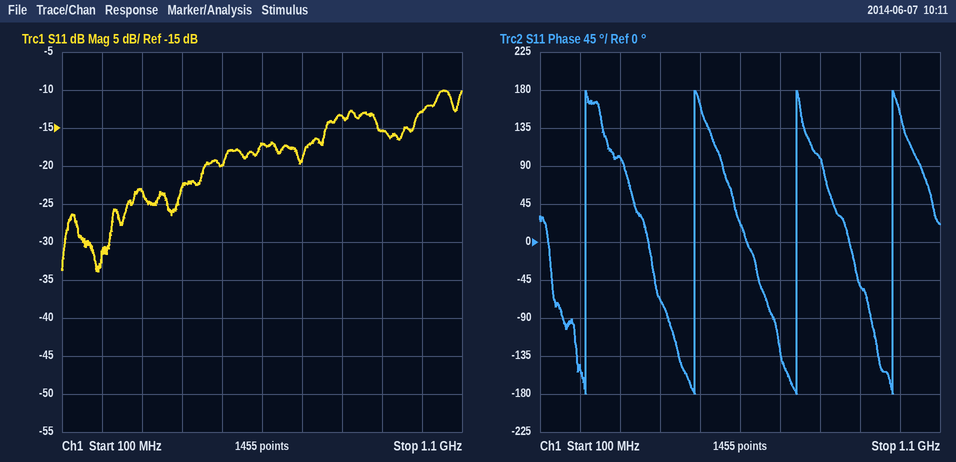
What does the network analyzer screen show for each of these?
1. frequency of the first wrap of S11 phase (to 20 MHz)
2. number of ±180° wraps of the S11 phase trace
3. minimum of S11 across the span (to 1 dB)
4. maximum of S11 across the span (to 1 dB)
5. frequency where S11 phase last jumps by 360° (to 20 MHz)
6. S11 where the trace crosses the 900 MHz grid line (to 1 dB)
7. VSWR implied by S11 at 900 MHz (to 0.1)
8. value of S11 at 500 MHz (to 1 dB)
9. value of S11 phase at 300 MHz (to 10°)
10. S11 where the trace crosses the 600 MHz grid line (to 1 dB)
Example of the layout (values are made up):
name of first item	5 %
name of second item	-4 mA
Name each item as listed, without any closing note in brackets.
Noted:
frequency of the first wrap of S11 phase	220 MHz
number of ±180° wraps of the S11 phase trace	4
minimum of S11 across the span	-34 dB
maximum of S11 across the span	-10 dB
frequency where S11 phase last jumps by 360°	980 MHz
S11 where the trace crosses the 900 MHz grid line	-15 dB
VSWR implied by S11 at 900 MHz	1.4
value of S11 at 500 MHz	-20 dB
value of S11 phase at 300 MHz	100°
S11 where the trace crosses the 600 MHz grid line	-17 dB
